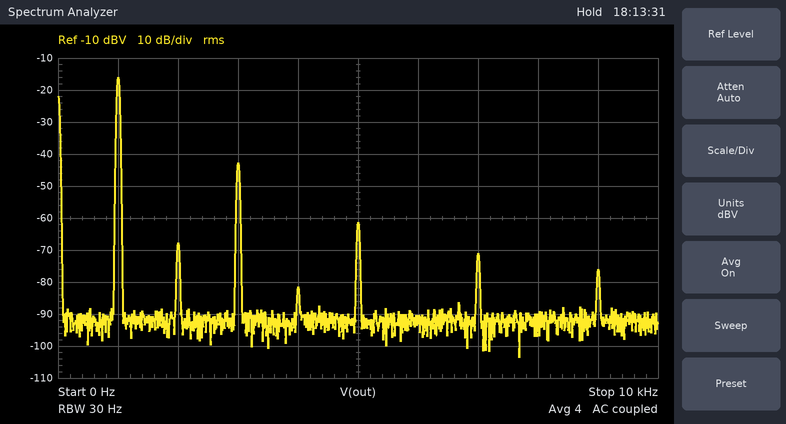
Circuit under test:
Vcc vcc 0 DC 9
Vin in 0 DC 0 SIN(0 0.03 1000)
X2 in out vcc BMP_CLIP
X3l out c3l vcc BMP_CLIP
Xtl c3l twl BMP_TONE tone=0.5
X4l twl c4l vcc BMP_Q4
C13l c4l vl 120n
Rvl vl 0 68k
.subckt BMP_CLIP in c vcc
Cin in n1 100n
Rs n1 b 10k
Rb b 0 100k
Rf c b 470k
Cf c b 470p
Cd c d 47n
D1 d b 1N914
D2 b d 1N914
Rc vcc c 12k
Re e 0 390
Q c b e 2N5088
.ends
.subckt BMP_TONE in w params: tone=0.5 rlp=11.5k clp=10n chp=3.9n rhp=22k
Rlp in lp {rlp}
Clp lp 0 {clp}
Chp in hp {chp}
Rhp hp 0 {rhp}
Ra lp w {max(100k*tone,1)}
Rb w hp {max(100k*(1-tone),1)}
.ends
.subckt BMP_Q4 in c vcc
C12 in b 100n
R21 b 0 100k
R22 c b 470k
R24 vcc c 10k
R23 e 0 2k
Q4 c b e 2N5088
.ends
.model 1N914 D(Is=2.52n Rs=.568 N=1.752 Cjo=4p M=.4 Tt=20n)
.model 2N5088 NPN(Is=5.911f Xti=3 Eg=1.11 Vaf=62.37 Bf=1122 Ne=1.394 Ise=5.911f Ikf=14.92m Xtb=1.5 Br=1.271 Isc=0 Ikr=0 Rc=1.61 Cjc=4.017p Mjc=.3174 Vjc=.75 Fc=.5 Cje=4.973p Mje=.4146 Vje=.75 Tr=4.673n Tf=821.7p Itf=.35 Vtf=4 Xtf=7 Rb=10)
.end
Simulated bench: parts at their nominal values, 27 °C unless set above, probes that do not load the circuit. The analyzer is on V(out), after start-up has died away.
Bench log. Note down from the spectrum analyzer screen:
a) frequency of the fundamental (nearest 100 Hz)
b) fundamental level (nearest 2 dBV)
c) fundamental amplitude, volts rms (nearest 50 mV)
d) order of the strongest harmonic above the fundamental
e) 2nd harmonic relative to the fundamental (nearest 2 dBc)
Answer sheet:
1.0 kHz
-16 dBV
150 mV
3
-52 dBc
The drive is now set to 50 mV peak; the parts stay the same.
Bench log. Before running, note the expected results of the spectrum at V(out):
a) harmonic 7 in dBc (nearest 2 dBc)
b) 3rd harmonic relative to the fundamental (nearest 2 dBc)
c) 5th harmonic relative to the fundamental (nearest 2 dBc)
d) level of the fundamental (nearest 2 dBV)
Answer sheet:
-46 dBc
-20 dBc
-36 dBc
-14 dBV
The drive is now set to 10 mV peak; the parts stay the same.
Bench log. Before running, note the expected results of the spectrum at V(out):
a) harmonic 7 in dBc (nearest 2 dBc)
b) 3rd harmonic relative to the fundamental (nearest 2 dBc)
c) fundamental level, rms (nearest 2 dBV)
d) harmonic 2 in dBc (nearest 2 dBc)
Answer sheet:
-56 dBc
-32 dBc
-24 dBV
-58 dBc
